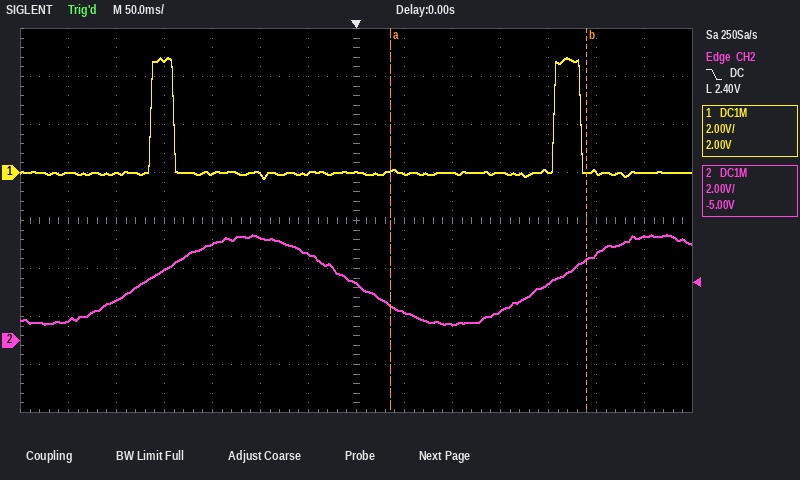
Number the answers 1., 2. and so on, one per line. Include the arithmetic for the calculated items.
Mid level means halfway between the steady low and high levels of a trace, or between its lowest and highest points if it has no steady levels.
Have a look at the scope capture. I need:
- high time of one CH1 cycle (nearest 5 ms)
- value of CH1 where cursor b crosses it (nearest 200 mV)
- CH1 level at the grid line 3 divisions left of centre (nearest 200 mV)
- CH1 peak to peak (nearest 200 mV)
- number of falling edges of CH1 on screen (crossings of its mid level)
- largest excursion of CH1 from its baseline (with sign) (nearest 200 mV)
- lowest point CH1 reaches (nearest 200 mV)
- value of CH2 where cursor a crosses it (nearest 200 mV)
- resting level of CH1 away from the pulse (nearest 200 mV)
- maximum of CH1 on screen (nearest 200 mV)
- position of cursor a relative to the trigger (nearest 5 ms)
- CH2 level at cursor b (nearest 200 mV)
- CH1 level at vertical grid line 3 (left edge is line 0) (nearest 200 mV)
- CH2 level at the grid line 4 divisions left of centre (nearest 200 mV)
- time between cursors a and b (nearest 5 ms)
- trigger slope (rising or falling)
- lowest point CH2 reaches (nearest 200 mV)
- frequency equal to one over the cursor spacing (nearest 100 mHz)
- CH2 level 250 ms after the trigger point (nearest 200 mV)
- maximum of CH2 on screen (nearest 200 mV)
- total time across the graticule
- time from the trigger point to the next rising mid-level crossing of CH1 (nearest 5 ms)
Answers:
1. 25 ms
2. 0.0 V
3. 0.0 V
4. 4.8 V − (-200 mV) = 5.0 V
5. 2
6. 4.8 V − (0.0 V) = +4.8 V
7. -200 mV
8. 1.4 V
9. 0.0 V
10. 4.8 V
11. +35 ms
12. 3.4 V
13. 4.6 V
14. 3.0 V
15. 205 ms
16. falling
17. 600 mV
18. 1 / 205 ms ≈ 4.9 Hz
19. 3.6 V
20. 4.4 V
21. 700 ms
22. 205 ms
